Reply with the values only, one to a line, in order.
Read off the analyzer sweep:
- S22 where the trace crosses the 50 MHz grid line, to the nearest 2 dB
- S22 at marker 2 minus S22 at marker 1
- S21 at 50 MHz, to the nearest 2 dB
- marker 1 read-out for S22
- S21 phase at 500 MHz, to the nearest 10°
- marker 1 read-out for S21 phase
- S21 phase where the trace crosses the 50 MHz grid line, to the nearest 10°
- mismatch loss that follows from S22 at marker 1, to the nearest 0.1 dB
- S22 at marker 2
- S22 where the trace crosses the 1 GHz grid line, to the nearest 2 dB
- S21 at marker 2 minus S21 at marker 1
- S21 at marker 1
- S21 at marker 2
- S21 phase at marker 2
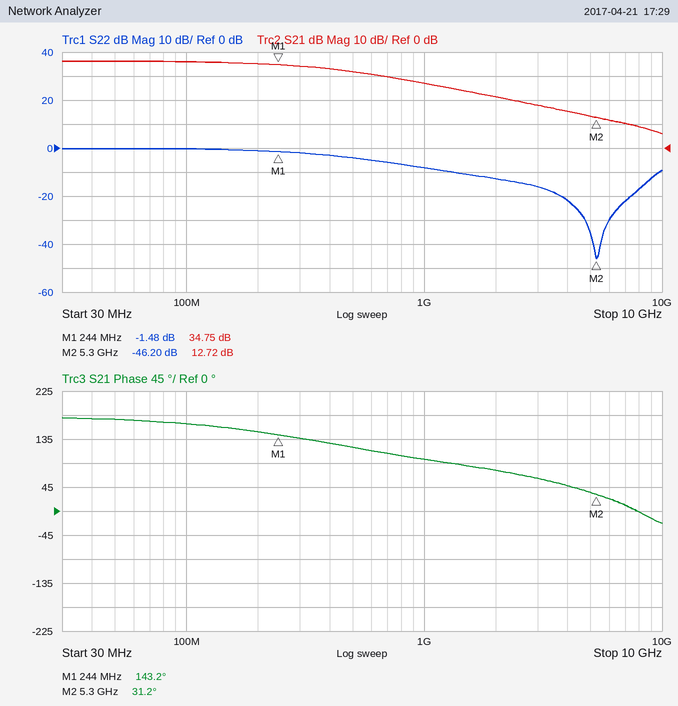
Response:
0 dB
-44.72 dB
36 dB
-1.48 dB
120°
143.2°
170°
5.4 dB
-46.20 dB
-8 dB
-22.03 dB
34.75 dB
12.72 dB
31.2°
